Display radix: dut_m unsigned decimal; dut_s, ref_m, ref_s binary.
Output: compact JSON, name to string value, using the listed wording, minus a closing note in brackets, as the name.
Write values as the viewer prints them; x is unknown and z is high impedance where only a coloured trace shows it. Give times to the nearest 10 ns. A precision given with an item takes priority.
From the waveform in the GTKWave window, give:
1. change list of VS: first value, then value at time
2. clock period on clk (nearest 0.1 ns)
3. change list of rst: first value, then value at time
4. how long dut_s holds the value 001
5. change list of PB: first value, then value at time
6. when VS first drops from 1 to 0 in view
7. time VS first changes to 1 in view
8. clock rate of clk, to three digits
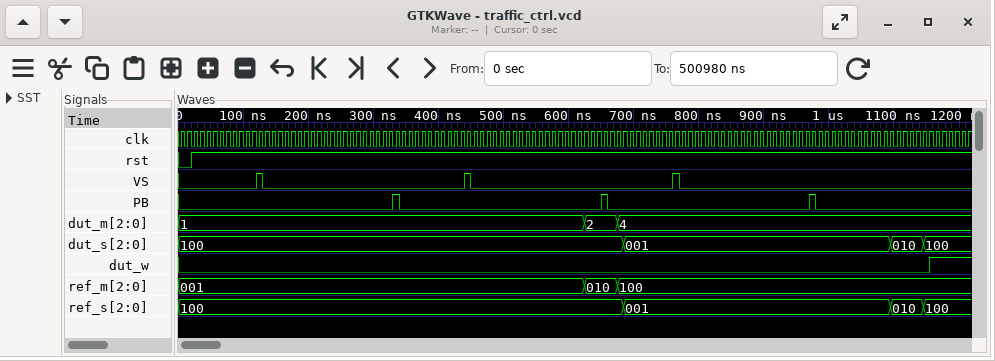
{"change list of VS: first value, then value at time": "0, 1 at 120 ns, 0 at 130 ns, 1 at 440 ns, 0 at 450 ns, 1 at 760 ns, 0 at 770 ns", "clock period on clk": "10 ns", "change list of rst: first value, then value at time": "0, 1 at 20 ns", "how long dut_s holds the value 001": "410 ns", "change list of PB: first value, then value at time": "0, 1 at 330 ns, 0 at 340 ns, 1 at 650 ns, 0 at 660 ns, 1 at 970 ns, 0 at 980 ns", "when VS first drops from 1 to 0 in view": "130 ns", "time VS first changes to 1 in view": "120 ns", "clock rate of clk, to three digits": "100 MHz"}
